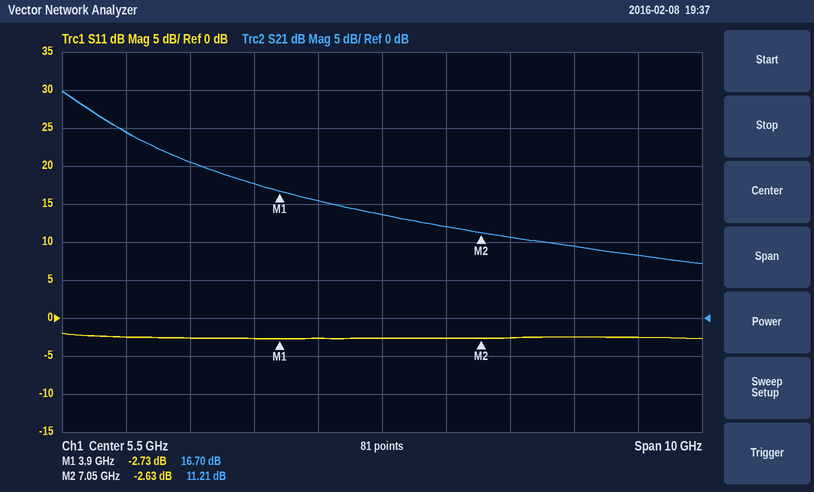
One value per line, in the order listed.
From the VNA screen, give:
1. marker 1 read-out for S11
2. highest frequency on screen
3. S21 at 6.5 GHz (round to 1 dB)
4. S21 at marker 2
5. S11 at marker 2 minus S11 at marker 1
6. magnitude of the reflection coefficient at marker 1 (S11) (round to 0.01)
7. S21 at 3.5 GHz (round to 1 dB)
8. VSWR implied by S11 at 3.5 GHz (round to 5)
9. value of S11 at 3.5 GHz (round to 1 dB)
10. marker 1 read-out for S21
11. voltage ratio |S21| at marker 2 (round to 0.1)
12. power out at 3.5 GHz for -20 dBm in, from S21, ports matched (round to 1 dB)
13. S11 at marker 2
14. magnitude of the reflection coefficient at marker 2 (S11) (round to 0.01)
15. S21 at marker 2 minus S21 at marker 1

-2.73 dB
10.5 GHz
12 dB
11.21 dB
0.10 dB
0.73
18 dB
5
-3 dB
16.70 dB
3.6
-2 dBm
-2.63 dB
0.74
-5.49 dB
